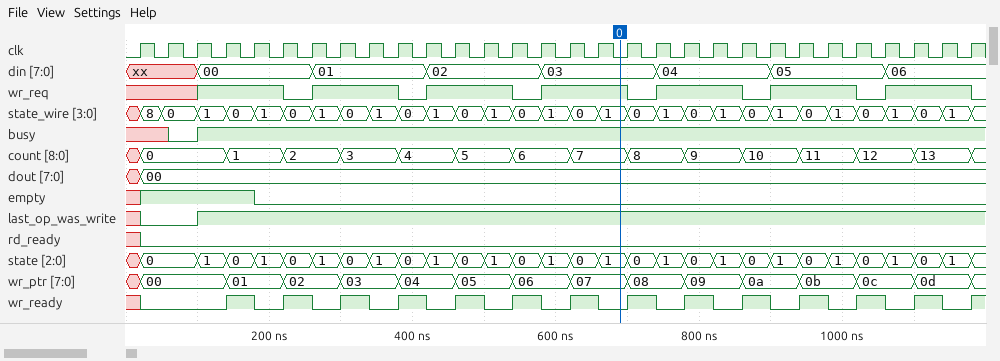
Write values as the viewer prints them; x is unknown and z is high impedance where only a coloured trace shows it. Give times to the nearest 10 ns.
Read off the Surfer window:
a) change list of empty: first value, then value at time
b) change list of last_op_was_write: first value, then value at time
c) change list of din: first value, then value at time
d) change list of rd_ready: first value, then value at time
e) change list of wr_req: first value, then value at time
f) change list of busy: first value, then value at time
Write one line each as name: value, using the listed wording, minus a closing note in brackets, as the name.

change list of empty: first value, then value at time: x, 1 at 20 ns, 0 at 180 ns
change list of last_op_was_write: first value, then value at time: x, 0 at 20 ns, 1 at 100 ns
change list of din: first value, then value at time: xx, 00 at 100 ns, 01 at 260 ns, 02 at 420 ns, 03 at 580 ns, 04 at 740 ns, 05 at 900 ns, 06 at 1060 ns
change list of rd_ready: first value, then value at time: x, 0 at 20 ns
change list of wr_req: first value, then value at time: x, 1 at 100 ns, 0 at 220 ns, 1 at 260 ns, 0 at 380 ns, 1 at 420 ns, 0 at 540 ns, 1 at 580 ns, 0 at 700 ns, 1 at 740 ns, 0 at 860 ns, 1 at 900 ns, 0 at 1020 ns, 1 at 1060 ns, 0 at 1180 ns
change list of busy: first value, then value at time: x, 0 at 60 ns, 1 at 100 ns
